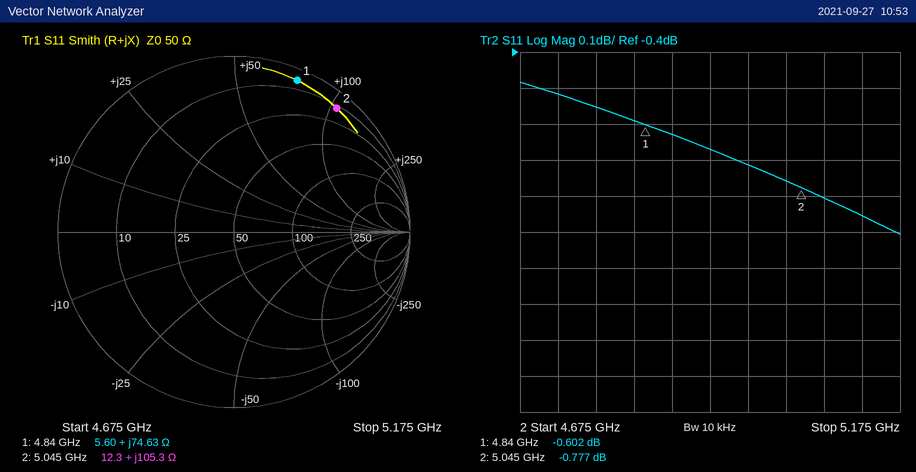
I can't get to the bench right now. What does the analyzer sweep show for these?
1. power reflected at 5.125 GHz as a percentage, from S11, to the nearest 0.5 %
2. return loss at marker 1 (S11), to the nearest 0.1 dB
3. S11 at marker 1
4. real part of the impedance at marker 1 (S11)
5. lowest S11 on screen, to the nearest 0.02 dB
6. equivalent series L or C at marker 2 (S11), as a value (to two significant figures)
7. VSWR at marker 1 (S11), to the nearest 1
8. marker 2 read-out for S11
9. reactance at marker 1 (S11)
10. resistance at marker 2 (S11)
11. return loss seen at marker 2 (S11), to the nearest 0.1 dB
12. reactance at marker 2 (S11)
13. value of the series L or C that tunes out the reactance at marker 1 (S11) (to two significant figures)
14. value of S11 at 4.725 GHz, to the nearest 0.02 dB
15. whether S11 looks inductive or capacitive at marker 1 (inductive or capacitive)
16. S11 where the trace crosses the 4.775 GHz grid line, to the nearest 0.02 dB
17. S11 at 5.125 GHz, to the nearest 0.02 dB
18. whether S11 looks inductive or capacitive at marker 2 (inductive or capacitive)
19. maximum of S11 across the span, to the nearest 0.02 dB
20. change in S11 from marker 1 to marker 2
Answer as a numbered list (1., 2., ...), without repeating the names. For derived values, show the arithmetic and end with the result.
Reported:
1. 10^(-0.86/10) ≈ 82.0 %
2. 0.6 dB
3. -0.602 dB
4. 5.60 Ω
5. -0.90 dB
6. L = 105.3 Ω/(2π × 5.045 GHz) ≈ 3.3 nH
7. (1 + 0.9330)/(1 − 0.9330) ≈ 29
8. -0.777 dB
9. +74.63 Ω
10. 12.3 Ω
11. 0.8 dB
12. +105.3 Ω
13. C = 1/(2π × 4.84 GHz × 74.63 Ω) ≈ 441 fF, so 440 fF to two significant figures
14. -0.52 dB
15. inductive
16. -0.56 dB
17. -0.86 dB
18. inductive
19. -0.48 dB
20. -0.777 − (-0.602) = -0.175 dB
